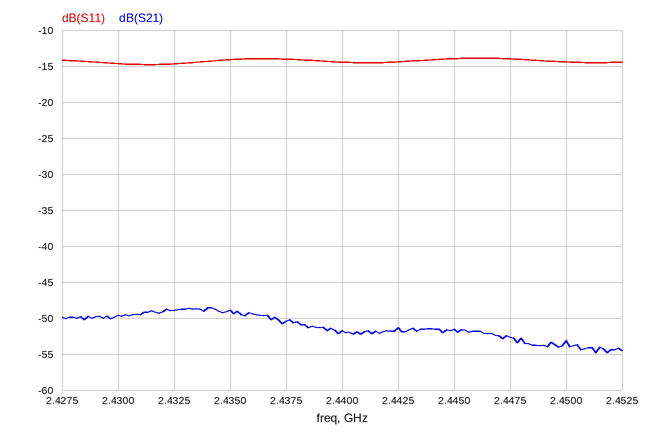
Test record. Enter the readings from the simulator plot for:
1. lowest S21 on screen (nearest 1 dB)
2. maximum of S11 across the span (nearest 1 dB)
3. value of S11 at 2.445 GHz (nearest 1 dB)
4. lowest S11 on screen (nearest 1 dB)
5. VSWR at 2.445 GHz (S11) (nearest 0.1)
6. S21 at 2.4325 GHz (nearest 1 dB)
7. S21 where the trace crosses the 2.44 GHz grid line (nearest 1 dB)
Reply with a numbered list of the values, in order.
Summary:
1. -55 dB
2. -14 dB
3. -14 dB
4. -15 dB
5. 1.5
6. -49 dB
7. -52 dB
